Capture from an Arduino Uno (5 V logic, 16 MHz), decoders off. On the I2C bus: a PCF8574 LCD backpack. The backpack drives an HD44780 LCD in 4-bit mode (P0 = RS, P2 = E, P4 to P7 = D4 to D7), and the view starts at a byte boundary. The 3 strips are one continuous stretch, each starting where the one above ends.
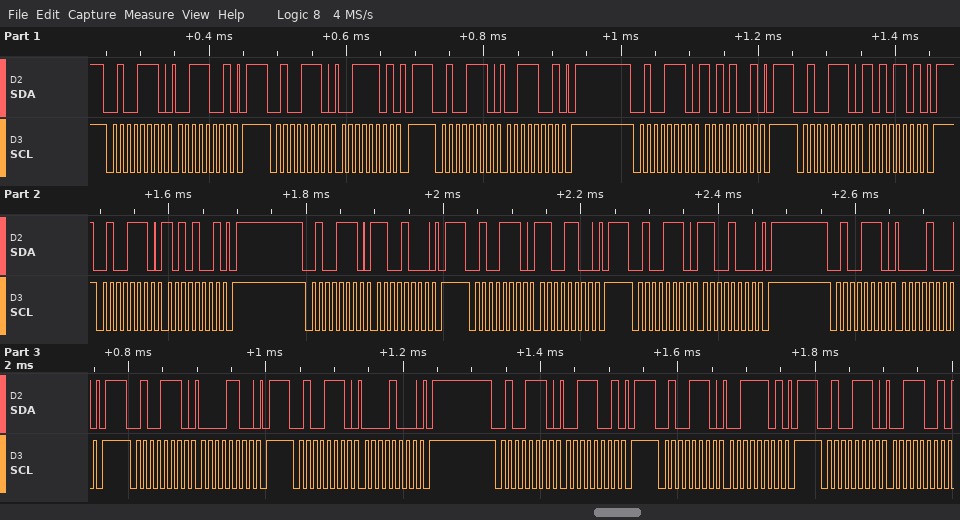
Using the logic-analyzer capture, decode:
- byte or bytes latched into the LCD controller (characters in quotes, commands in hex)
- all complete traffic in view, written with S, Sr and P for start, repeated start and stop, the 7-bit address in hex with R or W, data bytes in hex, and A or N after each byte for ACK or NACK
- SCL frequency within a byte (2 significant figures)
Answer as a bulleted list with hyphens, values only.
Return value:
- ':' 0xC0
- S 27W A 39 A P S 27W A 3D A P S 27W A 39 A P S 27W A A9 A P S 27W A AD A P S 27W A A9 A P S 27W A C8 A P S 27W A CC A P S 27W A C8 A P S 27W A 08 A P S 27W A 0C A P S 27W A 08 A P S 27W A 39 A P S 27W A 3D A P S 27W A 39 A
- 100 kHz
